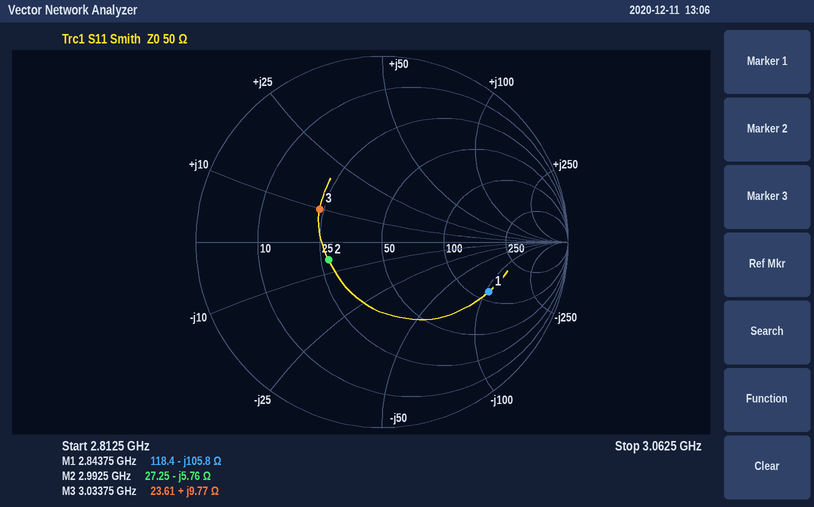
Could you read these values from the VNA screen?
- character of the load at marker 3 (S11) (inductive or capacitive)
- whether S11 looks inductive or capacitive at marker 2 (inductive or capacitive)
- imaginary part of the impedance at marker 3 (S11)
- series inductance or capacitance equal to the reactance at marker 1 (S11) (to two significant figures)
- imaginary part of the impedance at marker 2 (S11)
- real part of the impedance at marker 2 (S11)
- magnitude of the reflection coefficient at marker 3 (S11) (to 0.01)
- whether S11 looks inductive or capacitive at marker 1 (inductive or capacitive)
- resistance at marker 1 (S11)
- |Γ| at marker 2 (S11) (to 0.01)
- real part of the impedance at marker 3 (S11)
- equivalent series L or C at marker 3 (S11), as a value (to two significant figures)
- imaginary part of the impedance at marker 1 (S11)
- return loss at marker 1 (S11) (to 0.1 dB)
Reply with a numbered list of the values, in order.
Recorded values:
1. inductive
2. capacitive
3. +9.77 Ω
4. 530 fF
5. -5.76 Ω
6. 27.25 Ω
7. 0.38
8. capacitive
9. 118.4 Ω
10. 0.30
11. 23.61 Ω
12. 510 pH
13. -105.8 Ω
14. 4.0 dB
